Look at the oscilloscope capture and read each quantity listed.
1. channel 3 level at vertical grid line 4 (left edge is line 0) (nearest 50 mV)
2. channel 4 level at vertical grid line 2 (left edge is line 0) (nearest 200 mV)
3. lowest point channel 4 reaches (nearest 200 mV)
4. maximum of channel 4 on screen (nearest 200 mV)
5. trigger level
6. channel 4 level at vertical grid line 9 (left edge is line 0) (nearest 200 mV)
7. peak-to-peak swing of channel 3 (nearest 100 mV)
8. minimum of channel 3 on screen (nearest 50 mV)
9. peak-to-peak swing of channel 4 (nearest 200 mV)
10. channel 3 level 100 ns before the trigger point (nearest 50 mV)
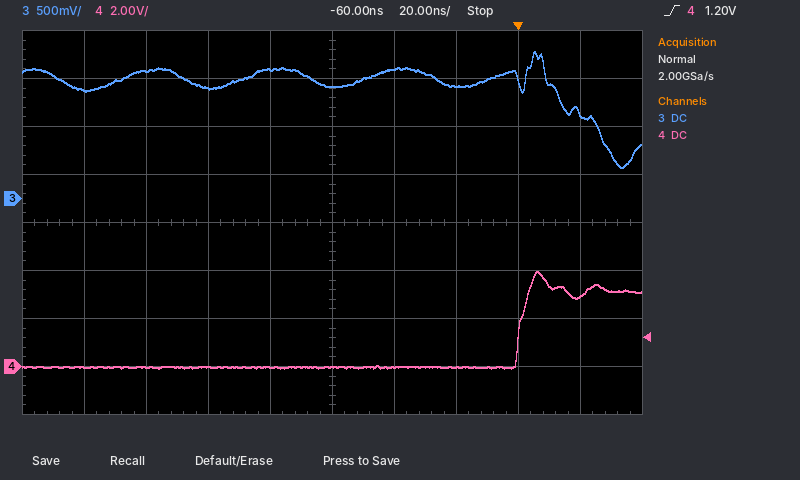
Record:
1.35 V
0.0 V
0.0 V
4.0 V
1.20 V
3.0 V
1.20 V
300 mV
4.0 V
1.15 V
